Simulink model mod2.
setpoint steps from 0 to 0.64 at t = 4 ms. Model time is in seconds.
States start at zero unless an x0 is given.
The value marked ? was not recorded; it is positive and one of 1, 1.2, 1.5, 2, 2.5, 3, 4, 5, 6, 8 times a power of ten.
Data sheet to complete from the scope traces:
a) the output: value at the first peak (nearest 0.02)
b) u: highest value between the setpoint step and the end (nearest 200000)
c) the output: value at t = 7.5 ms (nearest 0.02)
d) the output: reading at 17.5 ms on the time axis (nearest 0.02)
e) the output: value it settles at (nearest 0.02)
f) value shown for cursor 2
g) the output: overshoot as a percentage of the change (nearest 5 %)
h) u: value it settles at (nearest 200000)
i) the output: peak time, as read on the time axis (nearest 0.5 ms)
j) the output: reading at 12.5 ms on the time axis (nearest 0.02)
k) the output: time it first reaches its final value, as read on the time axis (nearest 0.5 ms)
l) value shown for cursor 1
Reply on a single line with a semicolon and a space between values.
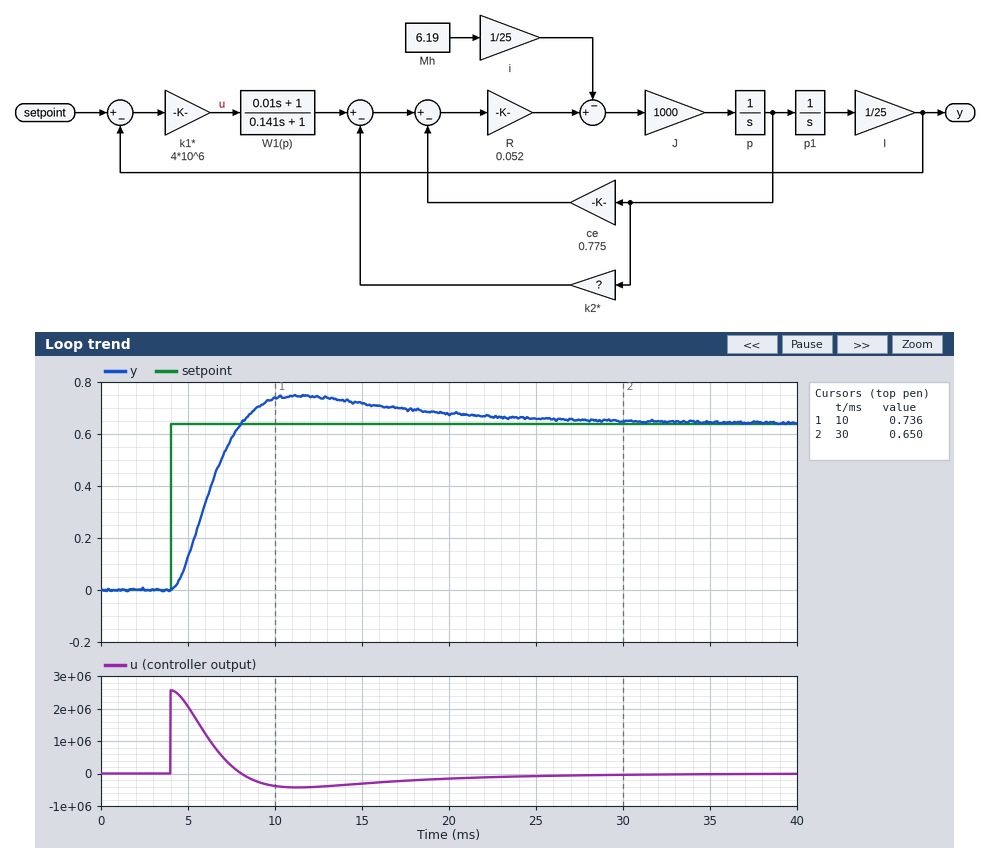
0.74; 2600000; 0.58; 0.70; 0.64; 0.650; 15 %; 0; 11.5 ms; 0.74; 8.0 ms; 0.736
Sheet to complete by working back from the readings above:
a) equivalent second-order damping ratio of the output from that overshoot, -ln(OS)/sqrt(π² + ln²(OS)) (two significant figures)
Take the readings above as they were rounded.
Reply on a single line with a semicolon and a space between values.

0.52
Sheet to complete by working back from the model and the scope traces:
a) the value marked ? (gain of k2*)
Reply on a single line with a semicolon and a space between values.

25
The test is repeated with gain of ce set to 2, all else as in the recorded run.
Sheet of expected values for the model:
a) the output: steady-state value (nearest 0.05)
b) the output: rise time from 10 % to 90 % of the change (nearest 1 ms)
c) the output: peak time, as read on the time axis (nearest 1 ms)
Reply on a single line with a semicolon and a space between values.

0.65; 3 ms; 12 ms
